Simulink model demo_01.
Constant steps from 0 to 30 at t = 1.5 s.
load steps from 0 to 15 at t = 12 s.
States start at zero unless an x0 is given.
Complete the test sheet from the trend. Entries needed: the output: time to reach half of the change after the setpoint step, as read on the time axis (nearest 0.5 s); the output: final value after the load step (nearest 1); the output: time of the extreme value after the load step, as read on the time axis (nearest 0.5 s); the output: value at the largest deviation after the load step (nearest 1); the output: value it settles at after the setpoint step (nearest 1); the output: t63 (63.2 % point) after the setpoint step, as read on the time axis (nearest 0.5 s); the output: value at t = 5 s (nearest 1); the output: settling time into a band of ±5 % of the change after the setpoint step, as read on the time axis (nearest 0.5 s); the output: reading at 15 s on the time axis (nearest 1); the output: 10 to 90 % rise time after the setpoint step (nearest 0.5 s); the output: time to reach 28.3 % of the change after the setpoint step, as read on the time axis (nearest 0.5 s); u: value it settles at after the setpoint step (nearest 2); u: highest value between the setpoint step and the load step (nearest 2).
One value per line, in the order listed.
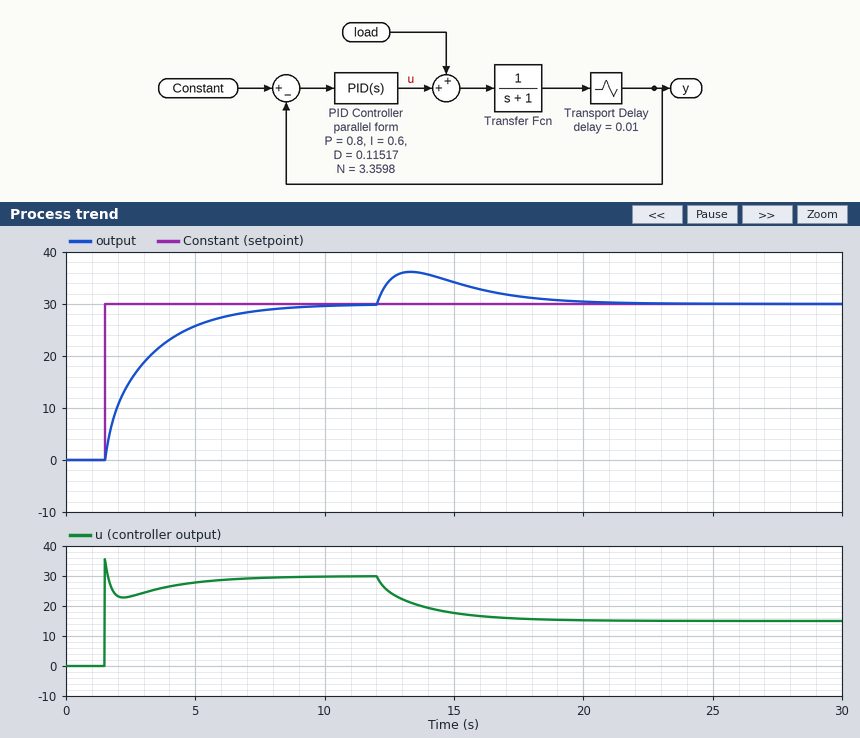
2.5 s
30
13.5 s
36
30
3.0 s
26
7.0 s
34
4.0 s
2.0 s
30
36
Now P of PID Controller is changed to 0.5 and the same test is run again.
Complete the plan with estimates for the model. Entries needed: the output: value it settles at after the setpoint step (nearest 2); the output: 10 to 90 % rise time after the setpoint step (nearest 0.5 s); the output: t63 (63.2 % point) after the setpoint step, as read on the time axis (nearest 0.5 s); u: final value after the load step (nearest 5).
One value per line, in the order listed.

30
3.5 s
3.5 s
15
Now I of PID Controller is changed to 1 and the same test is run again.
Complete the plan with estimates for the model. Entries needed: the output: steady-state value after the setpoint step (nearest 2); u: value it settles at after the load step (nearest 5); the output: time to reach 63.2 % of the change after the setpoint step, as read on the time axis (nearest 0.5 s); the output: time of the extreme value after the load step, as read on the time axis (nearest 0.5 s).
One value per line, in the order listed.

30
15
2.5 s
13.0 s
